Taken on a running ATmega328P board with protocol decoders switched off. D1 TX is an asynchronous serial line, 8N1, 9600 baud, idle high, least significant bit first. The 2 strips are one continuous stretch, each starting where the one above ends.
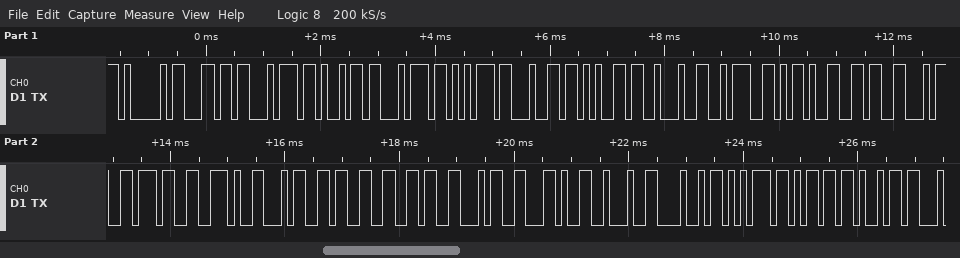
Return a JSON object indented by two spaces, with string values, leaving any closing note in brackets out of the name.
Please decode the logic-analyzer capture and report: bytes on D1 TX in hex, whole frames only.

{
  "bytes on D1 TX in hex, whole frames only": "41 6C 74 69 74 75 64 65 22 3A 2D 36 34 37 2E 34 33 36 34 2C 22 48 75 6D 69"
}
